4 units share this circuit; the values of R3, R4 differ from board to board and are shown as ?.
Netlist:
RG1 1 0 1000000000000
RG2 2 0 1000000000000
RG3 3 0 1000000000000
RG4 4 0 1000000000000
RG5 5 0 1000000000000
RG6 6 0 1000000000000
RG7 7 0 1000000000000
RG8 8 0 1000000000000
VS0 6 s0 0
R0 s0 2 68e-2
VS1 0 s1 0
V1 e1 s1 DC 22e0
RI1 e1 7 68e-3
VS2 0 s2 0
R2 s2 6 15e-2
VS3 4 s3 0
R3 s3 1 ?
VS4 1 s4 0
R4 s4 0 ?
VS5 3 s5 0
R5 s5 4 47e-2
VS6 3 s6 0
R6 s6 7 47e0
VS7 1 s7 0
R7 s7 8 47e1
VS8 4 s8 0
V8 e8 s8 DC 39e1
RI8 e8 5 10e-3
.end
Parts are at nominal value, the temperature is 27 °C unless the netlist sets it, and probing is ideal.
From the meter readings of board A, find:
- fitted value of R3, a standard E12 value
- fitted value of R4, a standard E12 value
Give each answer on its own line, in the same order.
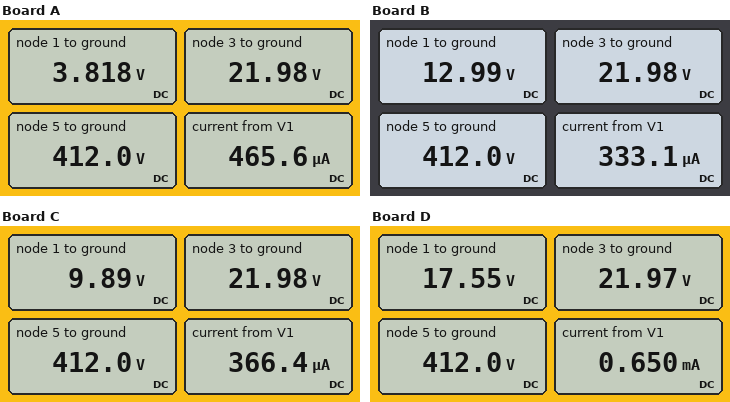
39 kΩ
8.2 kΩ
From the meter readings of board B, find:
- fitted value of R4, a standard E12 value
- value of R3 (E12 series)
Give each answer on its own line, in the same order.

39 kΩ
27 kΩ
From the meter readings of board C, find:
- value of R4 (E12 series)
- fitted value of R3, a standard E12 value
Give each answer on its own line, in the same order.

27 kΩ
33 kΩ
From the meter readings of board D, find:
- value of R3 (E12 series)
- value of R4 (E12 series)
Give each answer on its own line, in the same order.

6.8 kΩ
27 kΩ
